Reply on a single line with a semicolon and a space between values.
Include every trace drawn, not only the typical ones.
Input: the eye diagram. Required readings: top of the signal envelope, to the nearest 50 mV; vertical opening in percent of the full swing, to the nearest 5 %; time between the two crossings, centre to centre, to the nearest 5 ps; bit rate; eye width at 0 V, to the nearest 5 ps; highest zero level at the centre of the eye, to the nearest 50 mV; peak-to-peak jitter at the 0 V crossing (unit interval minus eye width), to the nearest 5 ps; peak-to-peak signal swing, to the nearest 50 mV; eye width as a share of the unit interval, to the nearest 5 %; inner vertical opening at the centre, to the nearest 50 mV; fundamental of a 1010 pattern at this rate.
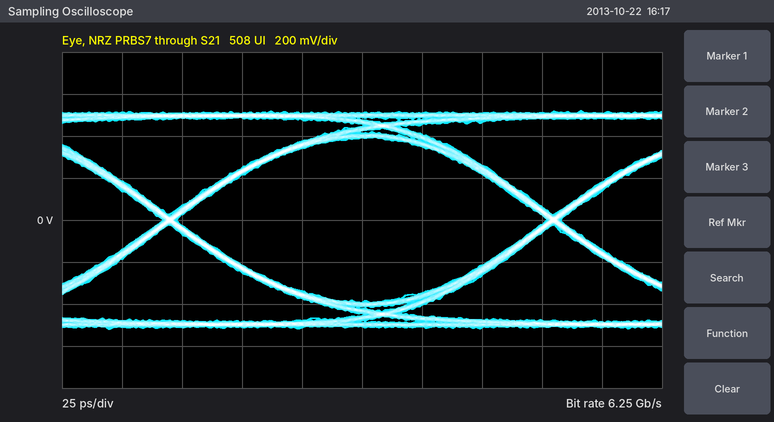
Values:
500 mV; 75 %; 160 ps; 6.25 Gb/s; 155 ps; -400 mV; 5 ps; 1.05 V; 95 %; 800 mV; 3.125 GHz
